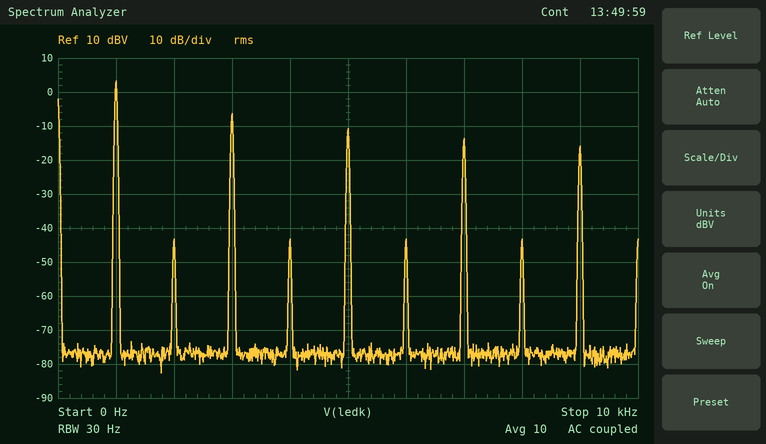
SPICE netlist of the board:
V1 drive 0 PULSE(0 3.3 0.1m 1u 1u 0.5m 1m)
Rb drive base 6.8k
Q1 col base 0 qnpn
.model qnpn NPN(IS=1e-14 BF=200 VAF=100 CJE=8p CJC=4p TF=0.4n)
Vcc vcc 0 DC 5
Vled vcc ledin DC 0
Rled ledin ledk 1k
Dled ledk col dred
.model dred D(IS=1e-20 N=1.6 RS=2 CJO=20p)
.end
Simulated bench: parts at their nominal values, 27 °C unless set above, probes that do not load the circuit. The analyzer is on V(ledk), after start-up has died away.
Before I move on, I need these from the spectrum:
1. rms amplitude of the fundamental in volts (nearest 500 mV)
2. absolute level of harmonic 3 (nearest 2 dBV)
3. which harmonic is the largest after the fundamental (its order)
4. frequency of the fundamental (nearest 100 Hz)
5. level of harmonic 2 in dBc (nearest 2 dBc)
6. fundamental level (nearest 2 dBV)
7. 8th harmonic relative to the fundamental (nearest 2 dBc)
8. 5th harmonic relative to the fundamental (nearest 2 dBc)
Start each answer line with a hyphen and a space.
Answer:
- 1.5 V
- -6 dBV
- 3
- 1.0 kHz
- -46 dBc
- 4 dBV
- -46 dBc
- -14 dBc
